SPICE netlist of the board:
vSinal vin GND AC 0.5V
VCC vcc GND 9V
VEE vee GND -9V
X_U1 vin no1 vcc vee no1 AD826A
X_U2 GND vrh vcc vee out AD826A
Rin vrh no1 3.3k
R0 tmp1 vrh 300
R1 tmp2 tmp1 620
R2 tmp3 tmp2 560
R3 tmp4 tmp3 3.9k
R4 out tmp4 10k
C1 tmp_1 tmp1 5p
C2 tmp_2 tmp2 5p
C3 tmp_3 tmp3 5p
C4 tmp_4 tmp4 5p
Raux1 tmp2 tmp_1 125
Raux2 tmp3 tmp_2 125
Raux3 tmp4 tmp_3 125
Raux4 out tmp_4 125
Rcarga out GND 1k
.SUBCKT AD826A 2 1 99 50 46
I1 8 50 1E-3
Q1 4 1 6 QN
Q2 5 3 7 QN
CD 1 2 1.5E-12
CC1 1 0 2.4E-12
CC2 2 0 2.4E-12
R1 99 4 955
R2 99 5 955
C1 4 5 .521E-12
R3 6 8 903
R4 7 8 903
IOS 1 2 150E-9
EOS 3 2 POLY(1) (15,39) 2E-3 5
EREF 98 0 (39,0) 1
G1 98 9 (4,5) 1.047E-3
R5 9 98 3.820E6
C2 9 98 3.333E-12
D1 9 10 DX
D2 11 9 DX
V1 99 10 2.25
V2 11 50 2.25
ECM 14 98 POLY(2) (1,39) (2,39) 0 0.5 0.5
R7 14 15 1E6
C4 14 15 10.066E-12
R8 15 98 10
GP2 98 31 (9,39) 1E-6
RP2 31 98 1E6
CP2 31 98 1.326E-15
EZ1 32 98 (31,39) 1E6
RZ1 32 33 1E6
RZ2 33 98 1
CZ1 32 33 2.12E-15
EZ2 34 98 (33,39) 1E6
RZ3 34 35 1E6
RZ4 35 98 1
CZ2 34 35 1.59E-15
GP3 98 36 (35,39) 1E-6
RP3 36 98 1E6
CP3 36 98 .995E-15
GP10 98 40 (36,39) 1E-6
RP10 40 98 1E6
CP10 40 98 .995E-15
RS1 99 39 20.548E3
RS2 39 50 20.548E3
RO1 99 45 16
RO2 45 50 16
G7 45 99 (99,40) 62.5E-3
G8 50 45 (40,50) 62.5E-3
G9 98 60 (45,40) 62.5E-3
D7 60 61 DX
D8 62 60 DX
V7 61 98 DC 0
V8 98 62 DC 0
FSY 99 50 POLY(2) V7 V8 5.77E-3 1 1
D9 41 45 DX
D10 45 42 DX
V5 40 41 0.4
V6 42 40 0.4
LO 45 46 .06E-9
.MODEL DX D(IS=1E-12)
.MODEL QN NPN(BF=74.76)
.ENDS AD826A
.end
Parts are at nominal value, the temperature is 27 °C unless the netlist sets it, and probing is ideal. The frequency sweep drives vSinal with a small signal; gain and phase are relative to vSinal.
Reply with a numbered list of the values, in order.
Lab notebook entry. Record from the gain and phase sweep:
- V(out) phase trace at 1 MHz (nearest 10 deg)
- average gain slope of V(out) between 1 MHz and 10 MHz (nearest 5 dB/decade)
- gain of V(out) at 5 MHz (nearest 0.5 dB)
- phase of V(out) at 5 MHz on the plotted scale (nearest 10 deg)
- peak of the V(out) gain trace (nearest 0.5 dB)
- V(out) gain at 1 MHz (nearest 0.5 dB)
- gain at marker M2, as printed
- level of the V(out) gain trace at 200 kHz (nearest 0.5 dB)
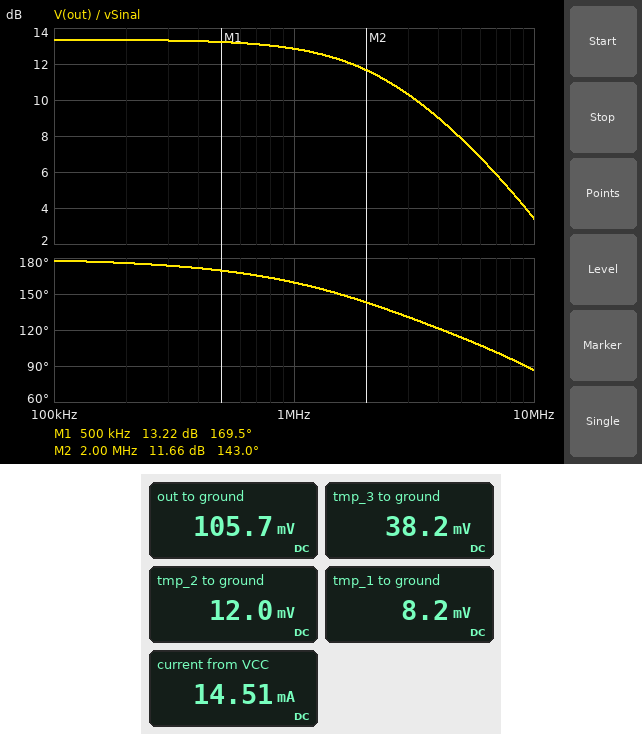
1. 160 deg
2. -10 dB/decade
3. 8.0 dB
4. 110 deg
5. 13.5 dB
6. 13.0 dB
7. 11.66 dB
8. 13.5 dB
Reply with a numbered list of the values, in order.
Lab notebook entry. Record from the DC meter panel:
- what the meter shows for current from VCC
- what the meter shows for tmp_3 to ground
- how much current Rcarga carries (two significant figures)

1. 14.51 mA
2. 38.2 mV
3. 110 µA
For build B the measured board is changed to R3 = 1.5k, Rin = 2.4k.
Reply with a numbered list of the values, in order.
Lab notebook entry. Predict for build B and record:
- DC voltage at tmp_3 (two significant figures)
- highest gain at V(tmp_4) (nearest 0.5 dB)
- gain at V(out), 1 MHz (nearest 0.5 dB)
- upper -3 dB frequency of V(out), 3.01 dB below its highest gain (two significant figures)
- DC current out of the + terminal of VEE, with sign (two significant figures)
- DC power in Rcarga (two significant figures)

1. 22 mV
2. 14.5 dB
3. 14.0 dB
4. 2.6 MHz
5. -14 mA
6. 8.0 µW
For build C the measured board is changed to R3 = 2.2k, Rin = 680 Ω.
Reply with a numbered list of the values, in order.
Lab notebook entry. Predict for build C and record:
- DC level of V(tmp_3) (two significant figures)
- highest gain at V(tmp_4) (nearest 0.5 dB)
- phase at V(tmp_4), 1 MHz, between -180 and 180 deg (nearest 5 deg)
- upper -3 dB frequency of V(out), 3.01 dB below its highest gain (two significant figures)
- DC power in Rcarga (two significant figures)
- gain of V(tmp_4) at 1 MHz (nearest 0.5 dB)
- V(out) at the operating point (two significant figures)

1. 27 mV
2. 26.0 dB
3. 145 deg
4. 1.5 MHz
5. 8.8 µW
6. 24.5 dB
7. 94 mV
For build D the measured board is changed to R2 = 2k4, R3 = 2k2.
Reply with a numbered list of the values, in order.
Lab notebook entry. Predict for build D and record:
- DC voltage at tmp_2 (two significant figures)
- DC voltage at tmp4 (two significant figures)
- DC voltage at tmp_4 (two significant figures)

1. 24 mV
2. 39 mV
3. 110 mV
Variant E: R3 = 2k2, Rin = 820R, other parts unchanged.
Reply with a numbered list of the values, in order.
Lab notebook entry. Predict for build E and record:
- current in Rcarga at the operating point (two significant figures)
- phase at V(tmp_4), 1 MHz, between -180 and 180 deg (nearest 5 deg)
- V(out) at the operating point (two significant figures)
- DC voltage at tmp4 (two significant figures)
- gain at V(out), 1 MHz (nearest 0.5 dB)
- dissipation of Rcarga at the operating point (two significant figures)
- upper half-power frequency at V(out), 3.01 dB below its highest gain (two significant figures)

1. 94 µA
2. 150 deg
3. 94 mV
4. 27 mV
5. 23.0 dB
6. 8.8 µW
7. 1.7 MHz
